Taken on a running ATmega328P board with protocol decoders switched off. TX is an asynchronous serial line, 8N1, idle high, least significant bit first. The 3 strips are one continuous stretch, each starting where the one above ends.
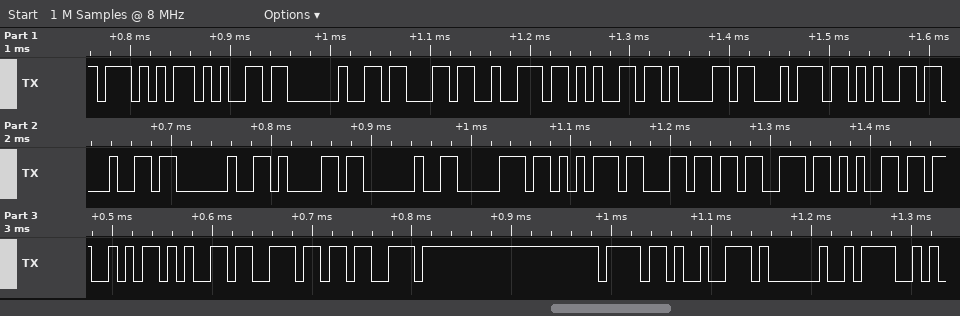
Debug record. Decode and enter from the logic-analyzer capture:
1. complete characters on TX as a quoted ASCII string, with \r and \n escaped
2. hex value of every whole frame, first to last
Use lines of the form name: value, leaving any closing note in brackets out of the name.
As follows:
complete characters on TX as a quoted ASCII string, with \r and \n escaped: "We created a pulseSensor O"
hex value of every whole frame, first to last: 57 65 20 63 72 65 61 74 65 64 20 61 20 70 75 6C 73 65 53 65 6E 73 6F 72 20 4F
